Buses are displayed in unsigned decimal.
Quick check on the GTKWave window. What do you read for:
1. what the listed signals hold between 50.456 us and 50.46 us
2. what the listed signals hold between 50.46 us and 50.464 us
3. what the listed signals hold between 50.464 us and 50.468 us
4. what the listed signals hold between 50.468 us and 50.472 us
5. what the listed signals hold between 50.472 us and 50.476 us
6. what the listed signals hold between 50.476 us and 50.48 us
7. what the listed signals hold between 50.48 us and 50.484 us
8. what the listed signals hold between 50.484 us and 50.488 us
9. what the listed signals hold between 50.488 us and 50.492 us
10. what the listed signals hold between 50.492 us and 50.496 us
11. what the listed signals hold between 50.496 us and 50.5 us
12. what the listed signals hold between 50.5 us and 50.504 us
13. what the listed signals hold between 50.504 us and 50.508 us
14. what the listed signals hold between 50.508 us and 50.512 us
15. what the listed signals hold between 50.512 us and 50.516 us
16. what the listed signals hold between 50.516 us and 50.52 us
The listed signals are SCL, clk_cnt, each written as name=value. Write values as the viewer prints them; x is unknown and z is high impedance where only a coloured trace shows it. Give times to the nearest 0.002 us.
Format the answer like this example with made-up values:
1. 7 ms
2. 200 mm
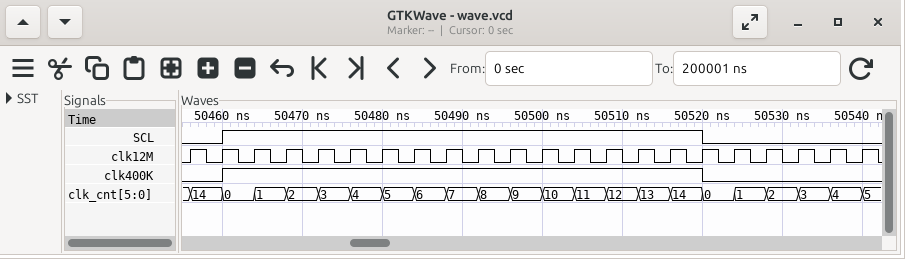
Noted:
1. SCL=0, clk_cnt=14
2. SCL=1, clk_cnt=0
3. SCL=1, clk_cnt=1
4. SCL=1, clk_cnt=2
5. SCL=1, clk_cnt=3
6. SCL=1, clk_cnt=4
7. SCL=1, clk_cnt=5
8. SCL=1, clk_cnt=6
9. SCL=1, clk_cnt=7
10. SCL=1, clk_cnt=8
11. SCL=1, clk_cnt=9
12. SCL=1, clk_cnt=10
13. SCL=1, clk_cnt=11
14. SCL=1, clk_cnt=12
15. SCL=1, clk_cnt=13
16. SCL=1, clk_cnt=14
